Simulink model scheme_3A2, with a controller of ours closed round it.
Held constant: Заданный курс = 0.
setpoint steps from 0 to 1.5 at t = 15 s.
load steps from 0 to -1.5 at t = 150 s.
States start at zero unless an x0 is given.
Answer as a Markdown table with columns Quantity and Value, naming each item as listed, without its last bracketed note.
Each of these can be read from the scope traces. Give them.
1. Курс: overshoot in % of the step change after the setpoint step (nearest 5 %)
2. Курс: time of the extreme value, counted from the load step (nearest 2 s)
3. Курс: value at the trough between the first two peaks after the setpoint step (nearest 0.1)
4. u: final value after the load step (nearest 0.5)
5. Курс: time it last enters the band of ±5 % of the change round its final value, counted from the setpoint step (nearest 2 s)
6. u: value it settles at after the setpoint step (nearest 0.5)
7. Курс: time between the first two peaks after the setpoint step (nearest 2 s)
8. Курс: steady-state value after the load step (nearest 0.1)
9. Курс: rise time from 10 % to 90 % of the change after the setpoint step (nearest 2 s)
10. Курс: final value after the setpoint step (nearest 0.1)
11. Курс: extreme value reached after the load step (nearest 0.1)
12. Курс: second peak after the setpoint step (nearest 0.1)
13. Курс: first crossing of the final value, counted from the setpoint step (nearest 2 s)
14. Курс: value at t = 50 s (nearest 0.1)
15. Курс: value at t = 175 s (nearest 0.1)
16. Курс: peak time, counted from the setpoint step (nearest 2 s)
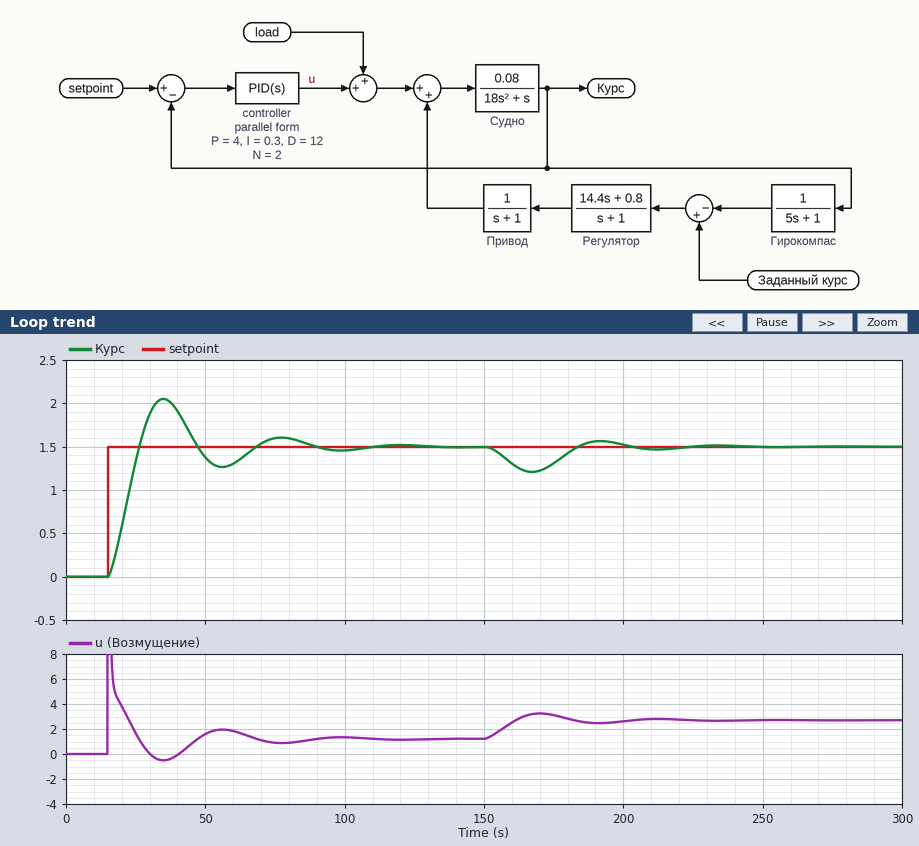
| Quantity | Value |
|---|---|
| Курс: overshoot in % of the step change after the setpoint step | 35 % |
| Курс: time of the extreme value, counted from the load step | 18 s |
| Курс: value at the trough between the first two peaks after the setpoint step | 1.3 |
| u: final value after the load step | 2.5 |
| Курс: time it last enters the band of ±5 % of the change round its final value, counted from the setpoint step | 68 s |
| u: value it settles at after the setpoint step | 1.0 |
| Курс: time between the first two peaks after the setpoint step | 42 s |
| Курс: steady-state value after the load step | 1.5 |
| Курс: rise time from 10 % to 90 % of the change after the setpoint step | 8 s |
| Курс: final value after the setpoint step | 1.5 |
| Курс: extreme value reached after the load step | 1.2 |
| Курс: second peak after the setpoint step | 1.6 |
| Курс: first crossing of the final value, counted from the setpoint step | 12 s |
| Курс: value at t = 50 s | 1.4 |
| Курс: value at t = 175 s | 1.3 |
| Курс: peak time, counted from the setpoint step | 20 s |
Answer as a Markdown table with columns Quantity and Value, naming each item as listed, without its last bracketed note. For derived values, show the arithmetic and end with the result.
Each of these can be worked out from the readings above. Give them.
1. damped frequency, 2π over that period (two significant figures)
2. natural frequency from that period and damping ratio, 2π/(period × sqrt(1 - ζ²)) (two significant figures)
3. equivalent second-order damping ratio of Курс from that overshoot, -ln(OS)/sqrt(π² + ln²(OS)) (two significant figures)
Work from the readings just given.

| Quantity | Value |
|---|---|
| damped frequency, 2π over that period | 2π / 42 = 0.15 rad/s |
| natural frequency from that period and damping ratio, 2π/(period × sqrt(1 - ζ²)) | 2π / (42 × sqrt(1 - 0.32²)) = 0.16 rad/s |
| equivalent second-order damping ratio of Курс from that overshoot, -ln(OS)/sqrt(π² + ln²(OS)) | ln(0.35) = -1.050; 1.050 / sqrt(9.870 + 1.102) = 0.32 |
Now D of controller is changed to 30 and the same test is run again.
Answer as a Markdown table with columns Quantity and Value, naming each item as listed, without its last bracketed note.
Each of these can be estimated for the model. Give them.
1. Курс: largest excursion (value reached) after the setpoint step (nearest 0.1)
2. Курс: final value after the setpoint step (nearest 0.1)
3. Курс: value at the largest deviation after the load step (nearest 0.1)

| Quantity | Value |
|---|---|
| Курс: largest excursion (value reached) after the setpoint step | 1.7 |
| Курс: final value after the setpoint step | 1.5 |
| Курс: value at the largest deviation after the load step | 1.3 |
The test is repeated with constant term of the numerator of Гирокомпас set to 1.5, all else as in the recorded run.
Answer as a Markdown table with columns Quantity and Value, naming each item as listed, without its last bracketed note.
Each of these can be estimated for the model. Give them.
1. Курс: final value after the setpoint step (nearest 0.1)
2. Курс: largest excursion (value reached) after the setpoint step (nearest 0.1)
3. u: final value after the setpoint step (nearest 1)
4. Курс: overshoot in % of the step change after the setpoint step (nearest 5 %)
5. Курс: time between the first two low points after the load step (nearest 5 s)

| Quantity | Value |
|---|---|
| Курс: final value after the setpoint step | 1.5 |
| Курс: largest excursion (value reached) after the setpoint step | 1.9 |
| u: final value after the setpoint step | 2 |
| Курс: overshoot in % of the step change after the setpoint step | 25 % |
| Курс: time between the first two low points after the load step | 40 s |
